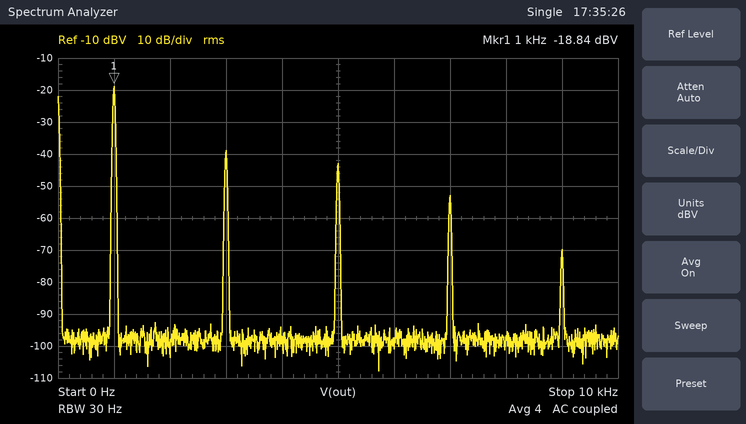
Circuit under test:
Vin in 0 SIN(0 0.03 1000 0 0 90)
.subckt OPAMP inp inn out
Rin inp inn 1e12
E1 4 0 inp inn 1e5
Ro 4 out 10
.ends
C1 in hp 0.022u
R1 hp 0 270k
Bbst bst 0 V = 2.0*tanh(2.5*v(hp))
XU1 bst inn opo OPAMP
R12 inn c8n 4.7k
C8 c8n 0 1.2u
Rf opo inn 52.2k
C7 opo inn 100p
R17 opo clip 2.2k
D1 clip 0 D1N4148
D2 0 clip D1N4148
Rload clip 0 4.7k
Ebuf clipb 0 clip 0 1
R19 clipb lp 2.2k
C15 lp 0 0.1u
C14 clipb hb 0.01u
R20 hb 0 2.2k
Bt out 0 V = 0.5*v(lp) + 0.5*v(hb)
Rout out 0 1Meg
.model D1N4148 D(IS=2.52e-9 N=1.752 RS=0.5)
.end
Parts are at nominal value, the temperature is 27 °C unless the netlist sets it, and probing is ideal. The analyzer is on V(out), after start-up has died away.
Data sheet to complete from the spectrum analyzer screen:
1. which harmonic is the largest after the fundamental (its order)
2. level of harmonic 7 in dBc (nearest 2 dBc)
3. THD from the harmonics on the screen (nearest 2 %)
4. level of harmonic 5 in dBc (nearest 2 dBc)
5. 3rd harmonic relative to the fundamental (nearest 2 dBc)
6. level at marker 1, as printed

3
-34 dBc
12 %
-24 dBc
-20 dBc
-18.84 dBV
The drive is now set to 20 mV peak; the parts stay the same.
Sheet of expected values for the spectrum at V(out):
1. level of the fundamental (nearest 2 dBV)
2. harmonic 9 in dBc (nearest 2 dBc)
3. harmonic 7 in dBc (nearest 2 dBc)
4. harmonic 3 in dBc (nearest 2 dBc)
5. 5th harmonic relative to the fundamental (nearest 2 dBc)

-20 dBV
-40 dBc
-40 dBc
-24 dBc
-36 dBc
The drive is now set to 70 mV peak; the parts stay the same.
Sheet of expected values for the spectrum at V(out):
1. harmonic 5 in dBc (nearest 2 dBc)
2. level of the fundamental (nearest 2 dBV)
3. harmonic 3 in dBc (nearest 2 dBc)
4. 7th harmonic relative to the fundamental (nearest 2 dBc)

-18 dBc
-18 dBV
-18 dBc
-20 dBc
